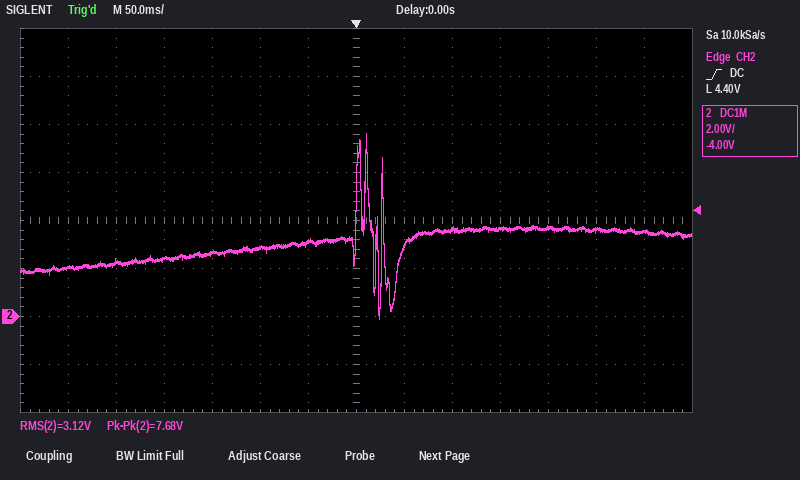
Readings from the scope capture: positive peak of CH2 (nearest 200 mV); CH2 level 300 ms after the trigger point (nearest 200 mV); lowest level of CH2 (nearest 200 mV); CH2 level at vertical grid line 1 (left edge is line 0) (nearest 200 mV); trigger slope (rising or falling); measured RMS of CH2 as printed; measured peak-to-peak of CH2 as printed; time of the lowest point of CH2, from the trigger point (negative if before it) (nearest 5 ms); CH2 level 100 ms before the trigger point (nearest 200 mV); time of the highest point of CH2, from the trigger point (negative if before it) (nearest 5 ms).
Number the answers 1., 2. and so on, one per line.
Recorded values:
1. 7.6 V
2. 3.6 V
3. 0.0 V
4. 2.0 V
5. rising
6. 3.12 V
7. 7.68 V
8. +25 ms
9. 2.8 V
10. +10 ms
